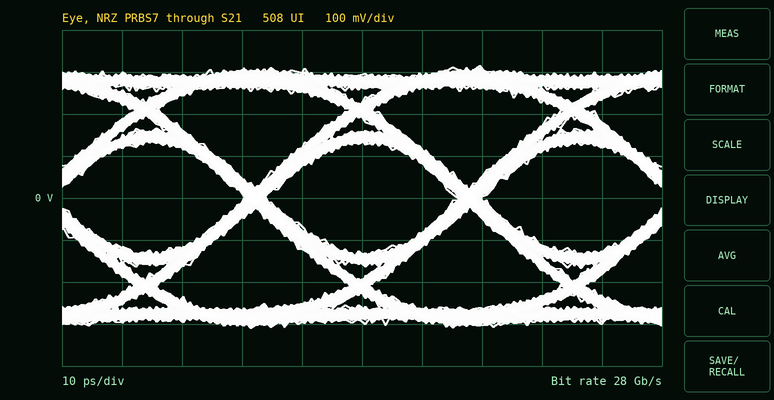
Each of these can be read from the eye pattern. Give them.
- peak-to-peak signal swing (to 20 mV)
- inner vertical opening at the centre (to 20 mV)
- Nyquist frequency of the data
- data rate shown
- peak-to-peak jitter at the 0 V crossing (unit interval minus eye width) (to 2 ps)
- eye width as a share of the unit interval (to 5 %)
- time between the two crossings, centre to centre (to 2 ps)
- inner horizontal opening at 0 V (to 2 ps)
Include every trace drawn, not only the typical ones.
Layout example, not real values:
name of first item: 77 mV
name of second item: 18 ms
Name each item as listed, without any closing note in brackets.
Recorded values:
peak-to-peak signal swing: 620 mV
inner vertical opening at the centre: 260 mV
Nyquist frequency of the data: 14 GHz
data rate shown: 28 Gb/s
peak-to-peak jitter at the 0 V crossing (unit interval minus eye width): 4 ps
eye width as a share of the unit interval: 90 %
time between the two crossings, centre to centre: 36 ps
inner horizontal opening at 0 V: 32 ps
